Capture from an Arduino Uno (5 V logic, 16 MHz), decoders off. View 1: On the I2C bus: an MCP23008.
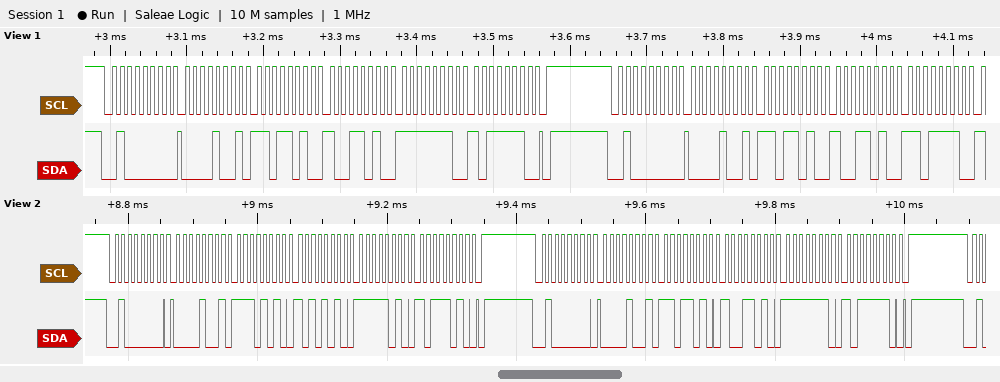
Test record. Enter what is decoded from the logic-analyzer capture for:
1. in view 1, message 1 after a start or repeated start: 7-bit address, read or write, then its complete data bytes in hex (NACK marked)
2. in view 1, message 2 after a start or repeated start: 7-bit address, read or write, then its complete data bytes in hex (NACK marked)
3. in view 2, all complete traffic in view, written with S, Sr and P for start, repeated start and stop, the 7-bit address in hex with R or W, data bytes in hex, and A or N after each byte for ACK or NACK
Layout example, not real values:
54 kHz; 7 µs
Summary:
0x20 write: 09 DA 9A FE BE; 0x20 write: 09 DA 9A DE; S 20W A 09 A EA A AA A FA A BA A P S 20W A 09 A DA A 9A A FE A BE A P
